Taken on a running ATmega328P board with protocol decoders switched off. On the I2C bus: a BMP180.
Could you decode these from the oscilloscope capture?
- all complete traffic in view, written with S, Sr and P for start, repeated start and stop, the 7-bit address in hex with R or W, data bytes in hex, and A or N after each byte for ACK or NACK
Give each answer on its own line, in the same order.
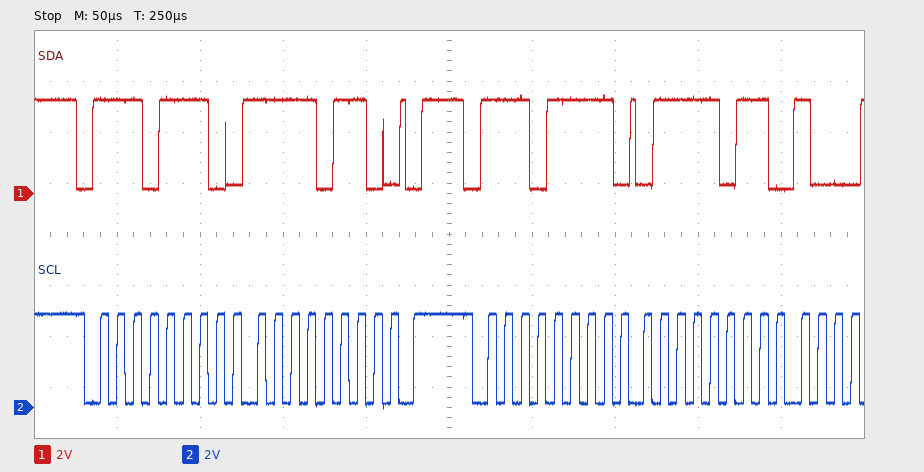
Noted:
S 77W A F6 A P S 77R A 7B A
